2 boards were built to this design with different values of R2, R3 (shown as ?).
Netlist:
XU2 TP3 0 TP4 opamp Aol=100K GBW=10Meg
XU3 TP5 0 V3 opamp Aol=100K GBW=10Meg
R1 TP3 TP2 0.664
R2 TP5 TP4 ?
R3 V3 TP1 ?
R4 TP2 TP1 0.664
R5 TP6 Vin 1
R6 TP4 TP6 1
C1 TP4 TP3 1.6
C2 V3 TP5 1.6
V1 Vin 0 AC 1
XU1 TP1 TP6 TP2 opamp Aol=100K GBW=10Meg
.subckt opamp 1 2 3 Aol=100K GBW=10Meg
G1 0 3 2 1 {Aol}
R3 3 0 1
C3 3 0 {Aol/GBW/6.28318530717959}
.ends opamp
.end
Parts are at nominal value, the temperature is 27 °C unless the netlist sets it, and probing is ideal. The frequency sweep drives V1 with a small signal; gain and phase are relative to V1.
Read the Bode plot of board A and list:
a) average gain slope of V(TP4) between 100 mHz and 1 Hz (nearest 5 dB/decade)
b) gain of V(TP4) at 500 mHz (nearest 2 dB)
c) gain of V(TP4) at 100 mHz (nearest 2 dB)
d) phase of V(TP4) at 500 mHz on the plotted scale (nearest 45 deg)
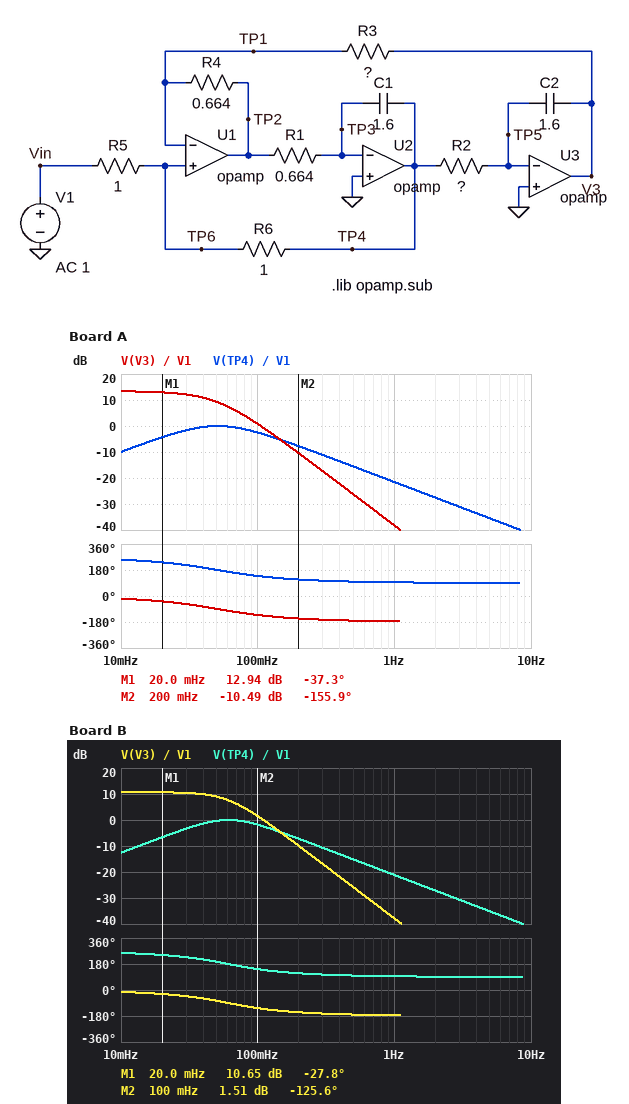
-20 dB/decade
-16 dB
-2 dB
90 deg
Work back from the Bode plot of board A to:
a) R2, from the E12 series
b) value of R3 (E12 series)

0.68 Ω
5.6 Ω
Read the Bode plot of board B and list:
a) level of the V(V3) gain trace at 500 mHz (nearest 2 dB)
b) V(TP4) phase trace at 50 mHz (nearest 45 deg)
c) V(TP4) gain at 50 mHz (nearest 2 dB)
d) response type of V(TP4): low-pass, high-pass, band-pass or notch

-26 dB
180 deg
0 dB
band-pass
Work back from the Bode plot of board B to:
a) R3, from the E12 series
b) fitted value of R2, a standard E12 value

3.9 Ω
0.68 Ω
